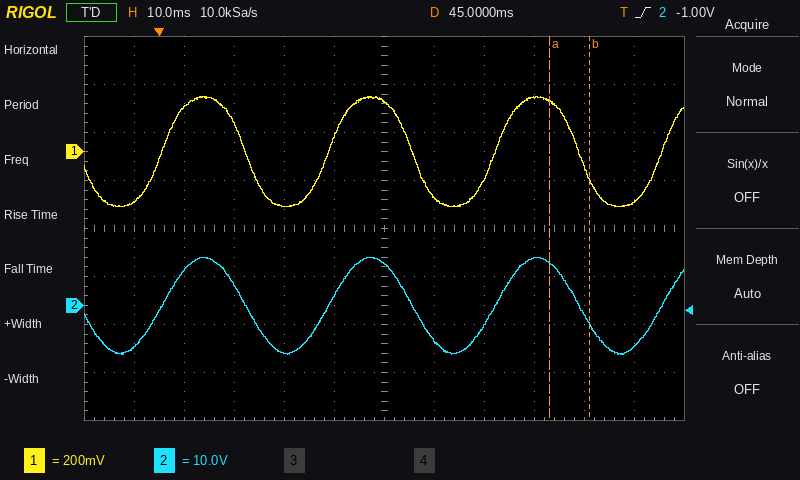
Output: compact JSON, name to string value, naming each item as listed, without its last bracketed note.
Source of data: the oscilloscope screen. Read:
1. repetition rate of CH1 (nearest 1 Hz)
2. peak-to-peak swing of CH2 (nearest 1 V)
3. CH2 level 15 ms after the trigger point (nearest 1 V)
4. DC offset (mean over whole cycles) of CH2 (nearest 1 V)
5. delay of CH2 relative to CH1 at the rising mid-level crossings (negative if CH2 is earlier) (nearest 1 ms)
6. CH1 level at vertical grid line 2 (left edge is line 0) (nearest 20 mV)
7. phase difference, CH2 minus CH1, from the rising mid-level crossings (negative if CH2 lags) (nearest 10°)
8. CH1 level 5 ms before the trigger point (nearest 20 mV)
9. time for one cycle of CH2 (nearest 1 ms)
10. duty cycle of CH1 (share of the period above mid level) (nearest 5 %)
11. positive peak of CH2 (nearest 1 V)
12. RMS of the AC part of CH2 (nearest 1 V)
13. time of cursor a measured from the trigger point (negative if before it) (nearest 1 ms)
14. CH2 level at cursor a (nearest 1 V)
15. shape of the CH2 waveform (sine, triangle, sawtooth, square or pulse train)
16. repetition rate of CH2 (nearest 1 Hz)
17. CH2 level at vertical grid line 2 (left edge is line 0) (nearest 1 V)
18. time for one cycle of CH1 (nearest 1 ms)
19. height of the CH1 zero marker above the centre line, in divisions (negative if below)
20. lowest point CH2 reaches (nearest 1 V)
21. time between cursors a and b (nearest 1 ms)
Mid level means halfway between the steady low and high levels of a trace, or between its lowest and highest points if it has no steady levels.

{"repetition rate of CH1": "30 Hz", "peak-to-peak swing of CH2": "20 V", "CH2 level 15 ms after the trigger point": "4 V", "DC offset (mean over whole cycles) of CH2": "0 V", "delay of CH2 relative to CH1 at the rising mid-level crossings (negative if CH2 is earlier)": "0 ms", "CH1 level at vertical grid line 2 (left edge is line 0)": "180 mV", "phase difference, CH2 minus CH1, from the rising mid-level crossings (negative if CH2 lags)": "0°", "CH1 level 5 ms before the trigger point": "-200 mV", "time for one cycle of CH2": "33 ms", "duty cycle of CH1 (share of the period above mid level)": "50 %", "positive peak of CH2": "10 V", "RMS of the AC part of CH2": "7 V", "time of cursor a measured from the trigger point (negative if before it)": "+78 ms", "CH2 level at cursor a": "9 V", "shape of the CH2 waveform": "sine", "repetition rate of CH2": "30 Hz", "CH2 level at vertical grid line 2 (left edge is line 0)": "7 V", "time for one cycle of CH1": "33 ms", "height of the CH1 zero marker above the centre line, in divisions": "+1.6 div", "lowest point CH2 reaches": "-10 V", "time between cursors a and b": "8 ms"}
